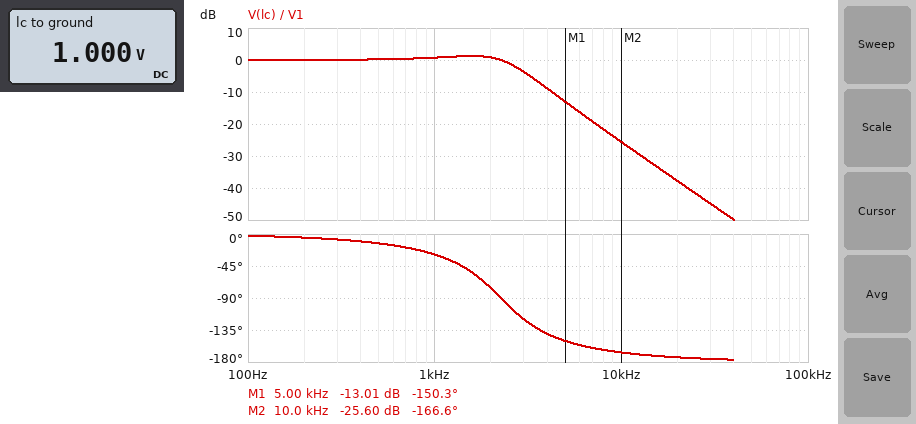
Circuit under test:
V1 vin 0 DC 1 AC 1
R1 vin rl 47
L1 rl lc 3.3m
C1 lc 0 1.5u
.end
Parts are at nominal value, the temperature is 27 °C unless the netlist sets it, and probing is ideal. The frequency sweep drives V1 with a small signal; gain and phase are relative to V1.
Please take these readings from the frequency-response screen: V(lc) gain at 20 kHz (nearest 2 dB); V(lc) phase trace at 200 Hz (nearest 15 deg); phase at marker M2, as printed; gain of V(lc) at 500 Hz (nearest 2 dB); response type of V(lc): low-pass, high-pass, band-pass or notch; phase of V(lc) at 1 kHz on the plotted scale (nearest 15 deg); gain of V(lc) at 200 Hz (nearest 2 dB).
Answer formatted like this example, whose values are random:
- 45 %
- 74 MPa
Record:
- -38 dB
- 0 deg
- -166.6 deg
- 0 dB
- low-pass
- -30 deg
- 0 dB
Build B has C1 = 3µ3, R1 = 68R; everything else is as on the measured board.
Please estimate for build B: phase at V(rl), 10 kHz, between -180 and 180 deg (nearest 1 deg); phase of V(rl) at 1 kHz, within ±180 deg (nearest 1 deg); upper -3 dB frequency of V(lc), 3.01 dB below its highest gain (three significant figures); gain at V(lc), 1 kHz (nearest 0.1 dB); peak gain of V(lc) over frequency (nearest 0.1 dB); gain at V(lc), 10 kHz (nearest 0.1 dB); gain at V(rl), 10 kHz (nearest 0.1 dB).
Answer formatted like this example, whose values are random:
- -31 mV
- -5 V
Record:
- 19 deg
- -68 deg
- 886 Hz
- -3.6 dB
- 0 dB
- -32.9 dB
- -0.5 dB
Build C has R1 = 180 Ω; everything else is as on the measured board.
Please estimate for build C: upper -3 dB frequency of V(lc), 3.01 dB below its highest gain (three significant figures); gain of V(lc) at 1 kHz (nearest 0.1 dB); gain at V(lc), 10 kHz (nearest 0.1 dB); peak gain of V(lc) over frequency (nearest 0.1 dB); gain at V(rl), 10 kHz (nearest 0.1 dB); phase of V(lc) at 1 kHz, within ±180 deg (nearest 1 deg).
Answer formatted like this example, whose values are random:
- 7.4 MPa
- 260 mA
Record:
- 632 Hz
- -5.5 dB
- -28.0 dB
- 0 dB
- -2.6 dB
- -65 deg
